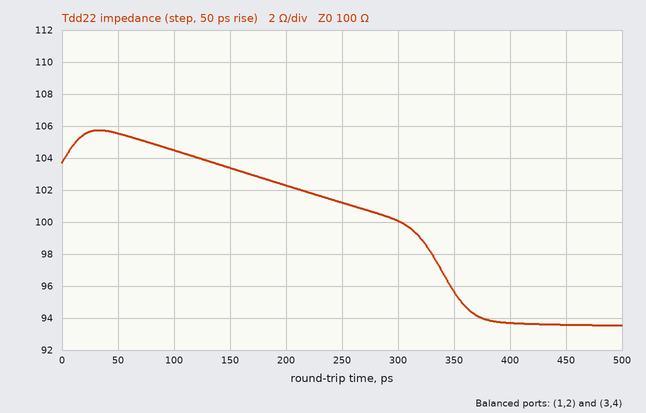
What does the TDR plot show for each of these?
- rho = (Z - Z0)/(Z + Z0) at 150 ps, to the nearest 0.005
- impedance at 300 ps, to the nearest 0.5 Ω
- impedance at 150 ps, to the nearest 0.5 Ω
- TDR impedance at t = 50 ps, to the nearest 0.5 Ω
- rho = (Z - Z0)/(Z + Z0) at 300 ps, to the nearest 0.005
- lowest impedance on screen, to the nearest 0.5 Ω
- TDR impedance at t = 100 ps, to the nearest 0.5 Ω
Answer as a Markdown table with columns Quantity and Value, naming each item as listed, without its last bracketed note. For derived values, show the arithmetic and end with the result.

| Quantity | Value |
|---|---|
| rho = (Z - Z0)/(Z + Z0) at 150 ps, to the nearest 0.005 | (103.5 − 100)/(103.5 + 100) ≈ +0.0172, so +0.015 to the nearest 0.005 |
| impedance at 300 ps, to the nearest 0.5 Ω | 100.0 Ω |
| impedance at 150 ps, to the nearest 0.5 Ω | 103.5 Ω |
| TDR impedance at t = 50 ps, to the nearest 0.5 Ω | 105.5 Ω |
| rho = (Z - Z0)/(Z + Z0) at 300 ps, to the nearest 0.005 | (100 − 100)/(100 + 100) ≈ 0.000 |
| lowest impedance on screen, to the nearest 0.5 Ω | 93.5 Ω |
| TDR impedance at t = 100 ps, to the nearest 0.5 Ω | 104.5 Ω |
